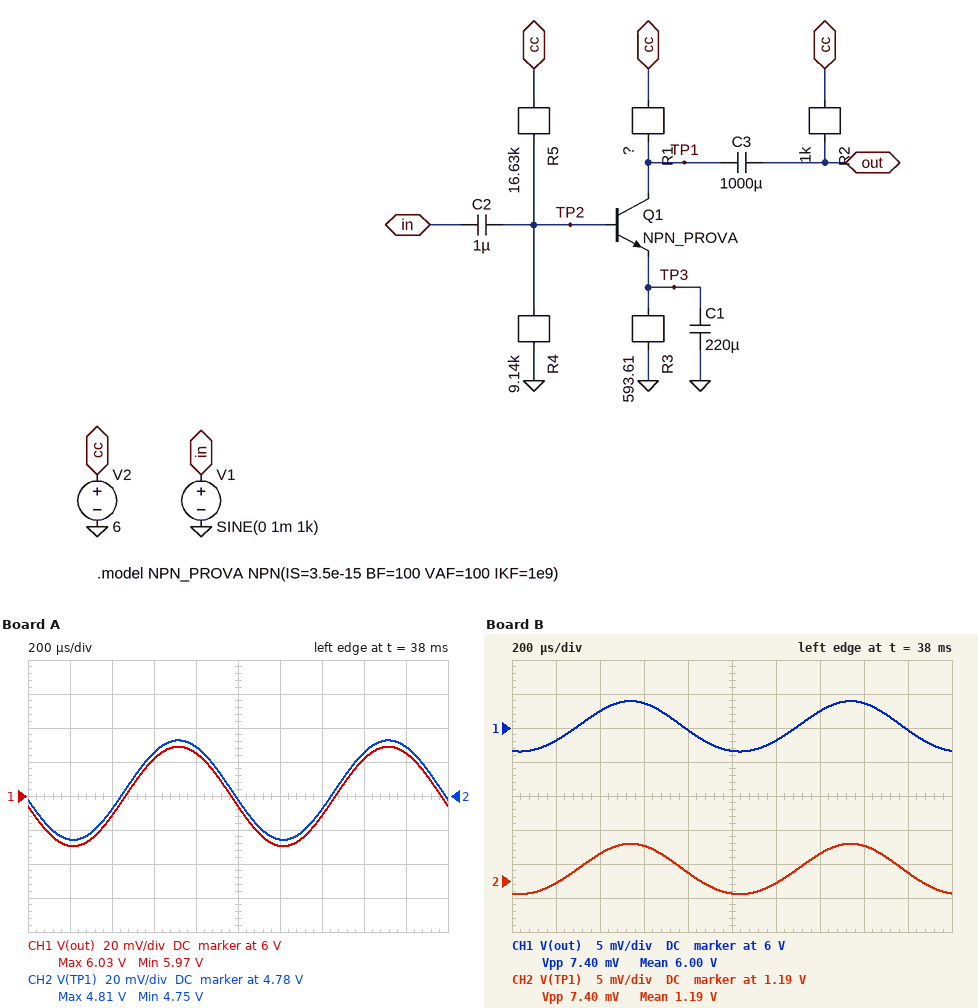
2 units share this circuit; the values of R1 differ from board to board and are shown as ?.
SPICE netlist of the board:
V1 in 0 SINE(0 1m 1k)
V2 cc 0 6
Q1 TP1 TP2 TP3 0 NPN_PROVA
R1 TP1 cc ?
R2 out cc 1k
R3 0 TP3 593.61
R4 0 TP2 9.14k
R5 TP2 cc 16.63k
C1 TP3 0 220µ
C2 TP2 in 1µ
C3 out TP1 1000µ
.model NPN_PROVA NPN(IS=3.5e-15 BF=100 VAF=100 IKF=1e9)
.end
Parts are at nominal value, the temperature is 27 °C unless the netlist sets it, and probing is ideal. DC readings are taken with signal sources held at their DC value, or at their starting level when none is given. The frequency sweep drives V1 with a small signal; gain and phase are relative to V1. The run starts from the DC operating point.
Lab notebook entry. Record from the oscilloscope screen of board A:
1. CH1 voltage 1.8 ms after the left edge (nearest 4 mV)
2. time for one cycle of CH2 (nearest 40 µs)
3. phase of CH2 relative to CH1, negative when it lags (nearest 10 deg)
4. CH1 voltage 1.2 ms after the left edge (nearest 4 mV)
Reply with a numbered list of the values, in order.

1. 6.024 V
2. 1.00 ms
3. 0 deg
4. 5.972 V
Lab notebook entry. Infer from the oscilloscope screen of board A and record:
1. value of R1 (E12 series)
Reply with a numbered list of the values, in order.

1. 560 Ω
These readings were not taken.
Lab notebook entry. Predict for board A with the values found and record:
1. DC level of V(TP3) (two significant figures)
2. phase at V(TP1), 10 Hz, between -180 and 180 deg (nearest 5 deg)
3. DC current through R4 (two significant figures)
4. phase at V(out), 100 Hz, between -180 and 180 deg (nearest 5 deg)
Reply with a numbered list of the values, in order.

1. 1.3 V
2. -60 deg
3. 220 µA
4. -110 deg
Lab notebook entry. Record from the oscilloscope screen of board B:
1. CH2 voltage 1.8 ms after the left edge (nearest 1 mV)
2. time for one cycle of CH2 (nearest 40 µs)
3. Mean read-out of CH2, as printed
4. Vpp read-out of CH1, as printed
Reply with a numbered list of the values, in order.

1. 1.191 V
2. 1.00 ms
3. 1.19 V
4. 7.40 mV
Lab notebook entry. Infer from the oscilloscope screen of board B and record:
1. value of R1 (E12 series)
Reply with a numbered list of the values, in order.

1. 2.7 kΩ
